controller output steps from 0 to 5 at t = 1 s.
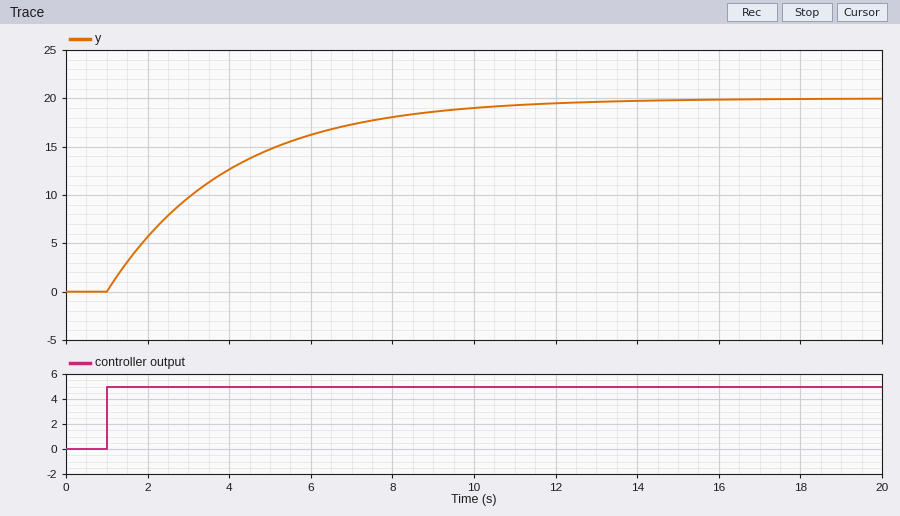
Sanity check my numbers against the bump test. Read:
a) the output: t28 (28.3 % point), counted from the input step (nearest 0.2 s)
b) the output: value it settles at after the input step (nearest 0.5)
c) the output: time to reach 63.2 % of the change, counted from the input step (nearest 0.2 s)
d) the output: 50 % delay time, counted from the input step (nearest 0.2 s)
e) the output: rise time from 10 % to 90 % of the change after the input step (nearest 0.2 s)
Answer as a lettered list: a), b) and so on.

a) 1.0 s
b) 20.0
c) 3.0 s
d) 2.0 s
e) 6.6 s
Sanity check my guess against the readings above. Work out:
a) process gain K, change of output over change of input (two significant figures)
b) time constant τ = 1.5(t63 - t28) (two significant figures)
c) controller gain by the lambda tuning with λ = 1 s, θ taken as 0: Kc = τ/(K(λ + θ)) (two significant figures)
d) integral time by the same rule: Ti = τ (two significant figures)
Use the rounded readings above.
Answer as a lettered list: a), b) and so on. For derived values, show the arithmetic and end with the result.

a) (20 - 0) / 5 = 4.0
b) 1.5 × (3 - 1) = 3.0 s
c) 3 / (4 × (1 + 0)) = 0.75
d) 3.0 s
